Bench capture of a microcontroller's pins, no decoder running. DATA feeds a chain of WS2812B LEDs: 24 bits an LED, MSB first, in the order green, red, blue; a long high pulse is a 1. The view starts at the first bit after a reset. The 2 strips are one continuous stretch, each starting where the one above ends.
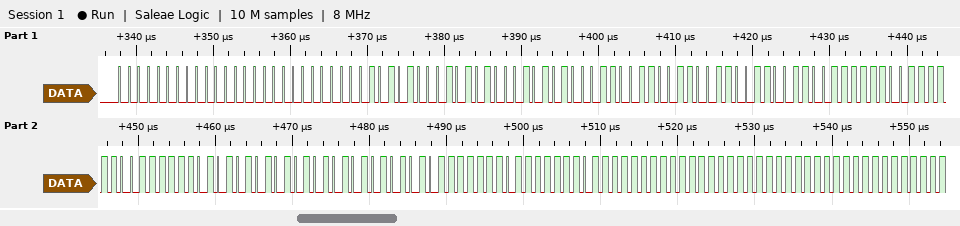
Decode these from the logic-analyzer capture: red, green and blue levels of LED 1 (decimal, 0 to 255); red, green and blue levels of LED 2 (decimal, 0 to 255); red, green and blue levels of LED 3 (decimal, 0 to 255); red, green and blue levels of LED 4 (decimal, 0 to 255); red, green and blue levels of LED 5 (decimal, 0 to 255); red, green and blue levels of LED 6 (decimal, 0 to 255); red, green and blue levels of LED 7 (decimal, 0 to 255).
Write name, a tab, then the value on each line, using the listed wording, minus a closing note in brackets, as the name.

red, green and blue levels of LED 1	0, 0, 0
red, green and blue levels of LED 2	42, 42, 42
red, green and blue levels of LED 3	51, 51, 51
red, green and blue levels of LED 4	63, 63, 63
red, green and blue levels of LED 5	85, 85, 85
red, green and blue levels of LED 6	127, 127, 127
red, green and blue levels of LED 7	255, 255, 255
